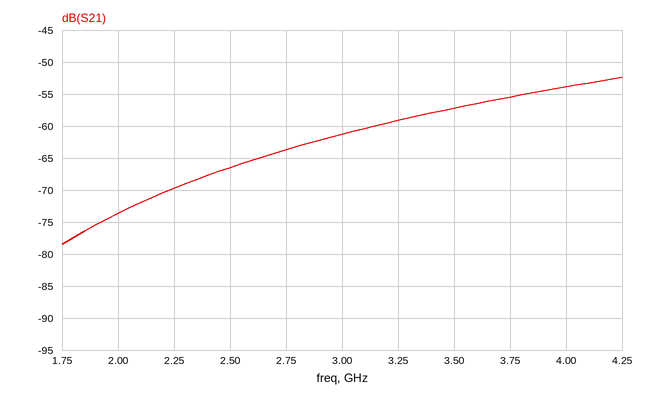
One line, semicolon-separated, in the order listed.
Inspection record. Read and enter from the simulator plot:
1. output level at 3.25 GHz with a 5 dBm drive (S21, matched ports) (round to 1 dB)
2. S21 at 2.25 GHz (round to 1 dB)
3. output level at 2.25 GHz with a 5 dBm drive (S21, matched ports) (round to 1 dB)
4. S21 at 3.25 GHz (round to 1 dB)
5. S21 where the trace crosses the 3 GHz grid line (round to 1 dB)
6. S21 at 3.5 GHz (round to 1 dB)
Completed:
-54 dBm; -70 dB; -65 dBm; -59 dB; -61 dB; -57 dB
